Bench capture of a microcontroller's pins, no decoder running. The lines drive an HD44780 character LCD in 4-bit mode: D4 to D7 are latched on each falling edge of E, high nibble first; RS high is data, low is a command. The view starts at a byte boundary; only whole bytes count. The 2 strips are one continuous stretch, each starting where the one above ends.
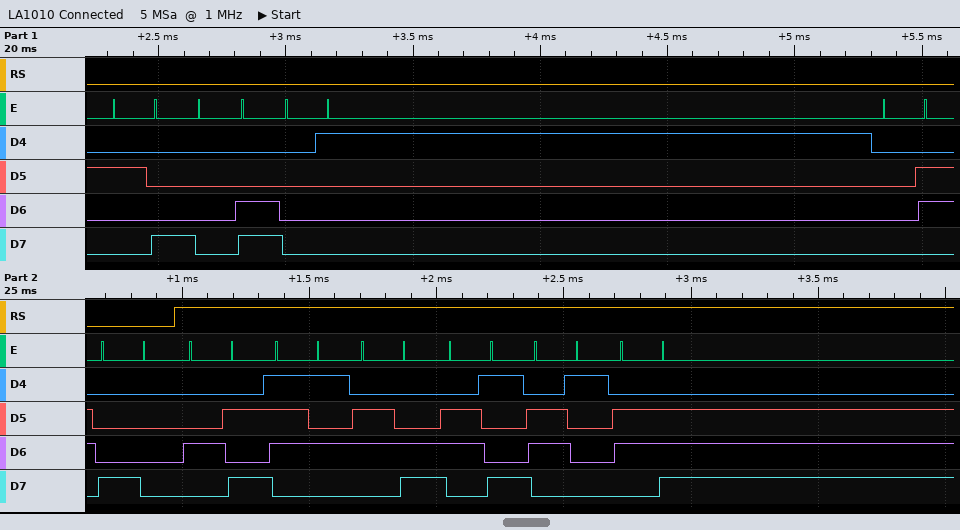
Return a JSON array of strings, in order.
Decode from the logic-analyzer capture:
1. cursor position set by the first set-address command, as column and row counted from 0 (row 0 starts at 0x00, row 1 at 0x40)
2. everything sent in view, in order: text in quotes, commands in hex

["column 0, row 0", "0x28 0x0C 0x01 0x06 0x80 \"Julian\""]
